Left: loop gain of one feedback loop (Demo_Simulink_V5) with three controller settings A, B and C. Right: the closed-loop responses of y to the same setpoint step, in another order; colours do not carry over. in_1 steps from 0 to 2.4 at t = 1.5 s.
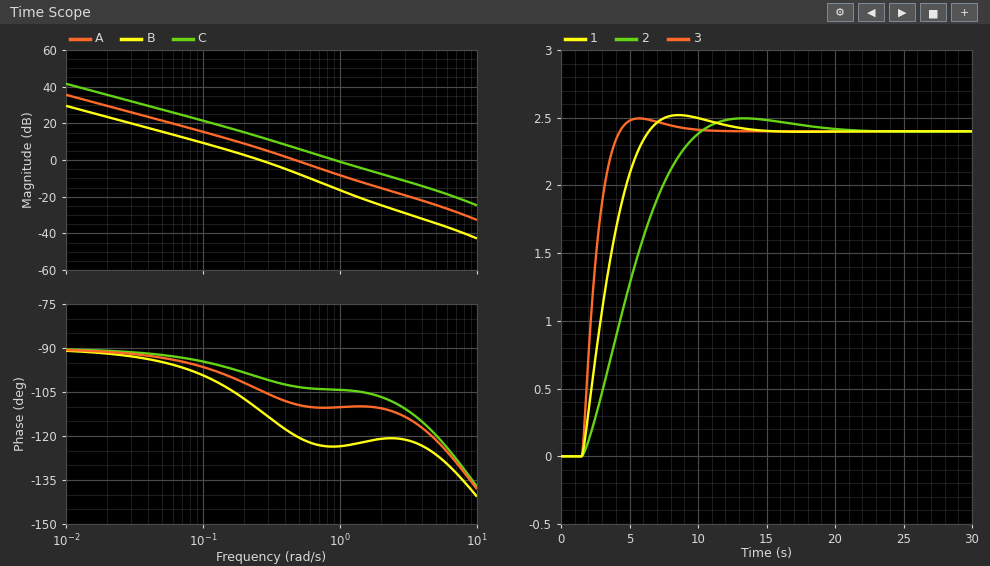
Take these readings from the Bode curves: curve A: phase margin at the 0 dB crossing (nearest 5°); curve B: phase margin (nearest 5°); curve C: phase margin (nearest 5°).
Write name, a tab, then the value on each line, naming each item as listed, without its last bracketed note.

curve A: phase margin at the 0 dB crossing	70°
curve B: phase margin	70°
curve C: phase margin	75°
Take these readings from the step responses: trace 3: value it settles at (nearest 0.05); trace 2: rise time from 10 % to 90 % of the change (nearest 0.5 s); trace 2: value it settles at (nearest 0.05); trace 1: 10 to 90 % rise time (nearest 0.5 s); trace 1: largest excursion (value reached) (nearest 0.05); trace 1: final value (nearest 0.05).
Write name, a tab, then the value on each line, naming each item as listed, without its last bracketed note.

trace 3: value it settles at	2.40
trace 2: rise time from 10 % to 90 % of the change	6.0 s
trace 2: value it settles at	2.40
trace 1: 10 to 90 % rise time	3.5 s
trace 1: largest excursion (value reached)	2.50
trace 1: final value	2.40
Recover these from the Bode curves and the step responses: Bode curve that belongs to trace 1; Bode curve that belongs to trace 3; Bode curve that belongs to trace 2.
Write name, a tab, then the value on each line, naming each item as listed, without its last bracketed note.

Bode curve that belongs to trace 1	A
Bode curve that belongs to trace 3	C
Bode curve that belongs to trace 2	B
